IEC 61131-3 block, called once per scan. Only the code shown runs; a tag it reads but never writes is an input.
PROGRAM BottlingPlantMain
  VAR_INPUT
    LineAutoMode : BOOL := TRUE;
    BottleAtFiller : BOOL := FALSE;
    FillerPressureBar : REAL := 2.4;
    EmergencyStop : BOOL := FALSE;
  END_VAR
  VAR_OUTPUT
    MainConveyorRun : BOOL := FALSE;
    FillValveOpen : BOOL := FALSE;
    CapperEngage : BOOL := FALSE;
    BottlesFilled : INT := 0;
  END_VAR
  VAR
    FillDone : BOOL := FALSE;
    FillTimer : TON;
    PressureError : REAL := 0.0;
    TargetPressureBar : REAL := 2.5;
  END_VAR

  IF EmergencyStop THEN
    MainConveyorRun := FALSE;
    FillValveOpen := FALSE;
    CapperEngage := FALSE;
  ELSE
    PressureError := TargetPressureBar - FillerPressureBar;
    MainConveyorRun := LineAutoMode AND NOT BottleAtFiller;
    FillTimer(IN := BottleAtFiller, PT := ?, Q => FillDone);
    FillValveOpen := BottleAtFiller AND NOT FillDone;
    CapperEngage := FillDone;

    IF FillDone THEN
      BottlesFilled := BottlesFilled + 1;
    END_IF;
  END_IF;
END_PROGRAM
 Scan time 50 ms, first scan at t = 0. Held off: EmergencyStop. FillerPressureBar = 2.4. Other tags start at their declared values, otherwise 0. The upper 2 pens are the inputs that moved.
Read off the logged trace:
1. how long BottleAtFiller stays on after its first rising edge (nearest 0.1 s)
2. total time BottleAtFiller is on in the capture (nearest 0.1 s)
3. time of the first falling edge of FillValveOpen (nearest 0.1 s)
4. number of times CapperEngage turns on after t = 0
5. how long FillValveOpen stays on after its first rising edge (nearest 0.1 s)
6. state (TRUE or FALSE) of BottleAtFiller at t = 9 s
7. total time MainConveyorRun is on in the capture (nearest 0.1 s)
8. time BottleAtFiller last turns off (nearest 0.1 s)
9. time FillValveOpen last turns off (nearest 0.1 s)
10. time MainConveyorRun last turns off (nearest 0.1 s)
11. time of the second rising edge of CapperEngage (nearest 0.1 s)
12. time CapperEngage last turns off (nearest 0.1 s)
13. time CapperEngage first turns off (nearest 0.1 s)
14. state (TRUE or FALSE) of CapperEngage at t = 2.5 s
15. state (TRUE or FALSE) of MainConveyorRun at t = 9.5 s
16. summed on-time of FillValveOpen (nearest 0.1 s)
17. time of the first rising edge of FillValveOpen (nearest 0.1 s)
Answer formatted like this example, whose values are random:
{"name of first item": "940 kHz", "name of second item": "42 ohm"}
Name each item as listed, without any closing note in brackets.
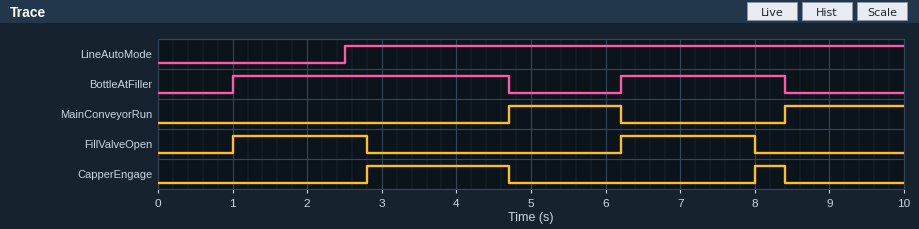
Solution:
{"how long BottleAtFiller stays on after its first rising edge": "3.7 s", "total time BottleAtFiller is on in the capture": "5.9 s", "time of the first falling edge of FillValveOpen": "2.8 s", "number of times CapperEngage turns on after t = 0": "2", "how long FillValveOpen stays on after its first rising edge": "1.8 s", "state (TRUE or FALSE) of BottleAtFiller at t = 9 s": "FALSE", "total time MainConveyorRun is on in the capture": "3.1 s", "time BottleAtFiller last turns off": "8.4 s", "time FillValveOpen last turns off": "8.0 s", "time MainConveyorRun last turns off": "6.2 s", "time of the second rising edge of CapperEngage": "8.0 s", "time CapperEngage last turns off": "8.4 s", "time CapperEngage first turns off": "4.7 s", "state (TRUE or FALSE) of CapperEngage at t = 2.5 s": "FALSE", "state (TRUE or FALSE) of MainConveyorRun at t = 9.5 s": "TRUE", "summed on-time of FillValveOpen": "3.6 s", "time of the first rising edge of FillValveOpen": "1.0 s"}
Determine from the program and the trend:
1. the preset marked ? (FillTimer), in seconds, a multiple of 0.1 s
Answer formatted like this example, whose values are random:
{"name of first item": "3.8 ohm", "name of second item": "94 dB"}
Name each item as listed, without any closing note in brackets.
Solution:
{"the preset marked ? (FillTimer), in seconds, a multiple of 0.1 s": "1.8 s"}
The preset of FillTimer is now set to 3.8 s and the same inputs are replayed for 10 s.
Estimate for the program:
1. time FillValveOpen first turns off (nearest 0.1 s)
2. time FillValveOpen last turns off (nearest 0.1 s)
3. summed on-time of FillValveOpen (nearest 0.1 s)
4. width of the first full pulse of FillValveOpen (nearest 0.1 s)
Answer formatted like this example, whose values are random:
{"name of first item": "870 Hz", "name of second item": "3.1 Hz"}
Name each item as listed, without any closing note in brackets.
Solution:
{"time FillValveOpen first turns off": "4.7 s", "time FillValveOpen last turns off": "8.4 s", "summed on-time of FillValveOpen": "5.9 s", "width of the first full pulse of FillValveOpen": "3.7 s"}
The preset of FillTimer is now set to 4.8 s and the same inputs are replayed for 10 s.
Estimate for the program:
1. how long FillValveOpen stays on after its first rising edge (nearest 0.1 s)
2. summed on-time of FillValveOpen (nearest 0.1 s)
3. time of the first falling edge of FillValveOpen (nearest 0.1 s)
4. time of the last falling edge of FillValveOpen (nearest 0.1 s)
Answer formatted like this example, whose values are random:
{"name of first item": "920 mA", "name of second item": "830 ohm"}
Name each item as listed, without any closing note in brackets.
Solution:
{"how long FillValveOpen stays on after its first rising edge": "3.7 s", "summed on-time of FillValveOpen": "5.9 s", "time of the first falling edge of FillValveOpen": "4.7 s", "time of the last falling edge of FillValveOpen": "8.4 s"}
